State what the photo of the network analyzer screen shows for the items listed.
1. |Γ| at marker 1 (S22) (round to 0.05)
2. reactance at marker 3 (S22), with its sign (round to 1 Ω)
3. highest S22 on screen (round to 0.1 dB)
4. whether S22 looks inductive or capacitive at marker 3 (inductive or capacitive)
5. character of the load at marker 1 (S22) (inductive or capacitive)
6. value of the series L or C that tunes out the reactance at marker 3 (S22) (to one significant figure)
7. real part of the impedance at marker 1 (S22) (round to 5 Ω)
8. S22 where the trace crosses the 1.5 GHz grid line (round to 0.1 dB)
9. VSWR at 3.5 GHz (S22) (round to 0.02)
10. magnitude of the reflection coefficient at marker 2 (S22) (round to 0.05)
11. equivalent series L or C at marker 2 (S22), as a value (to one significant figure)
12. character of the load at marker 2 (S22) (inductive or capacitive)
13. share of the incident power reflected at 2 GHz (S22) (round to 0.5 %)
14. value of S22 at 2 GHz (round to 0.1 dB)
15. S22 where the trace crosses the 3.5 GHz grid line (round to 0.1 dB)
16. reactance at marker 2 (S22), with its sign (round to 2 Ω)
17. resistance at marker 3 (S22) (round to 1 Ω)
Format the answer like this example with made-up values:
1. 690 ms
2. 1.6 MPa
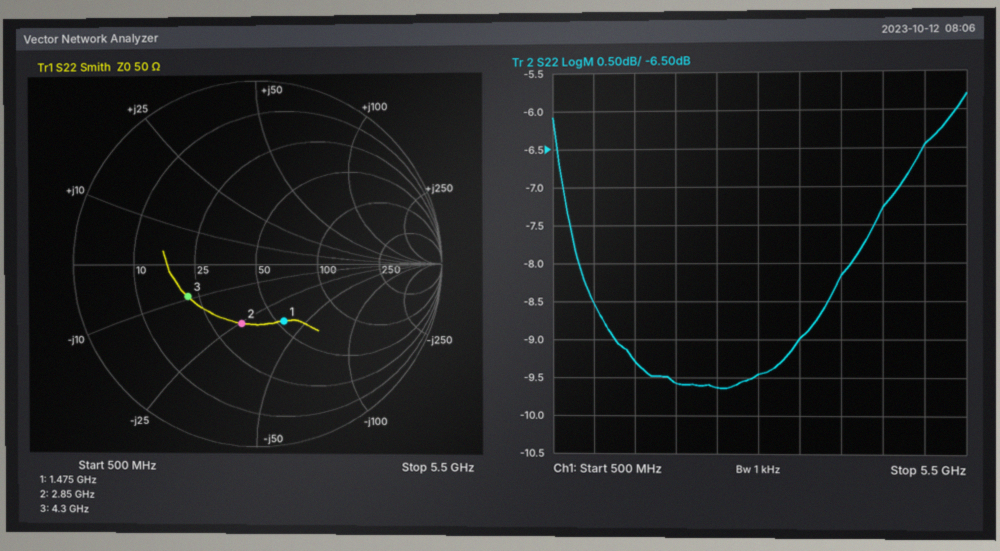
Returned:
1. 0.35
2. -9 Ω
3. -5.8 dB
4. capacitive
5. capacitive
6. 300 pH
7. 55 Ω
8. -9.3 dB
9. 2.10
10. 0.35
11. 2 pF
12. capacitive
13. 11.0 %
14. -9.6 dB
15. -9.0 dB
16. -26 Ω
17. 22 Ω
